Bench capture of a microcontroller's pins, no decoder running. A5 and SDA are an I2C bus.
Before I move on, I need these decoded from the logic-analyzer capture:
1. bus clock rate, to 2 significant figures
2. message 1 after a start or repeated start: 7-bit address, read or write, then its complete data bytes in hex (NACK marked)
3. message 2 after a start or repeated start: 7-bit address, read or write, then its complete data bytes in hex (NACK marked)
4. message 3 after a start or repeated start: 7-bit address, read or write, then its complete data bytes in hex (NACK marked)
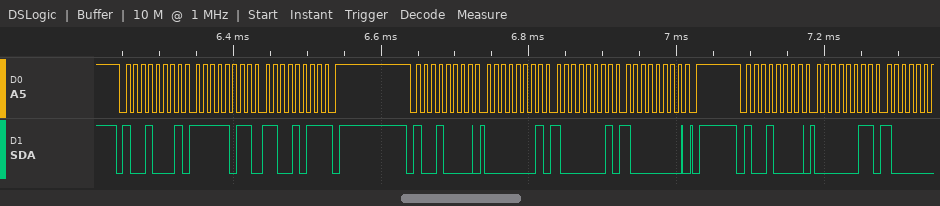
100 kHz
0x48 read: FB CB NACK
0x48 write: 01 81 80
0x48 write: 03
